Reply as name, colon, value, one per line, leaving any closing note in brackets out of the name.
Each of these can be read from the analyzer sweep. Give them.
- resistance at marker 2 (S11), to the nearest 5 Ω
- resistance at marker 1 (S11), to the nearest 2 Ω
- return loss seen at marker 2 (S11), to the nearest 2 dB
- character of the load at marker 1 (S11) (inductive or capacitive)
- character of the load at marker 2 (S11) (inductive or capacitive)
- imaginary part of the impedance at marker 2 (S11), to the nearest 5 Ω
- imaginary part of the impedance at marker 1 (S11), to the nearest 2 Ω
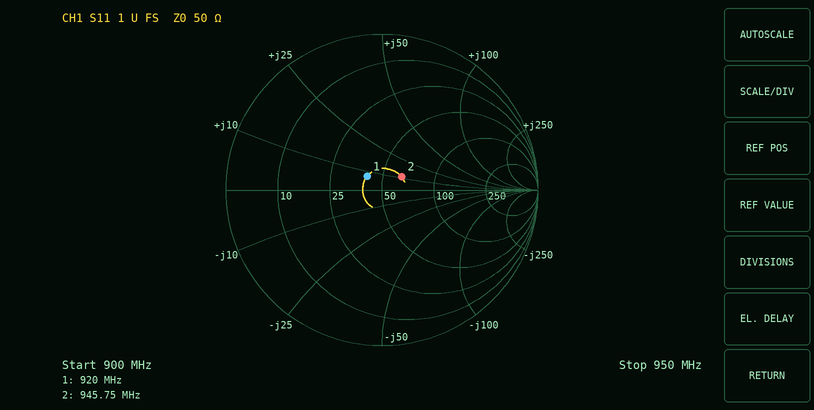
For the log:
resistance at marker 2 (S11), to the nearest 5 Ω: 65 Ω
resistance at marker 1 (S11), to the nearest 2 Ω: 40 Ω
return loss seen at marker 2 (S11), to the nearest 2 dB: 16 dB
character of the load at marker 1 (S11): inductive
character of the load at marker 2 (S11): inductive
imaginary part of the impedance at marker 2 (S11), to the nearest 5 Ω: +10 Ω
imaginary part of the impedance at marker 1 (S11), to the nearest 2 Ω: +8 Ω
